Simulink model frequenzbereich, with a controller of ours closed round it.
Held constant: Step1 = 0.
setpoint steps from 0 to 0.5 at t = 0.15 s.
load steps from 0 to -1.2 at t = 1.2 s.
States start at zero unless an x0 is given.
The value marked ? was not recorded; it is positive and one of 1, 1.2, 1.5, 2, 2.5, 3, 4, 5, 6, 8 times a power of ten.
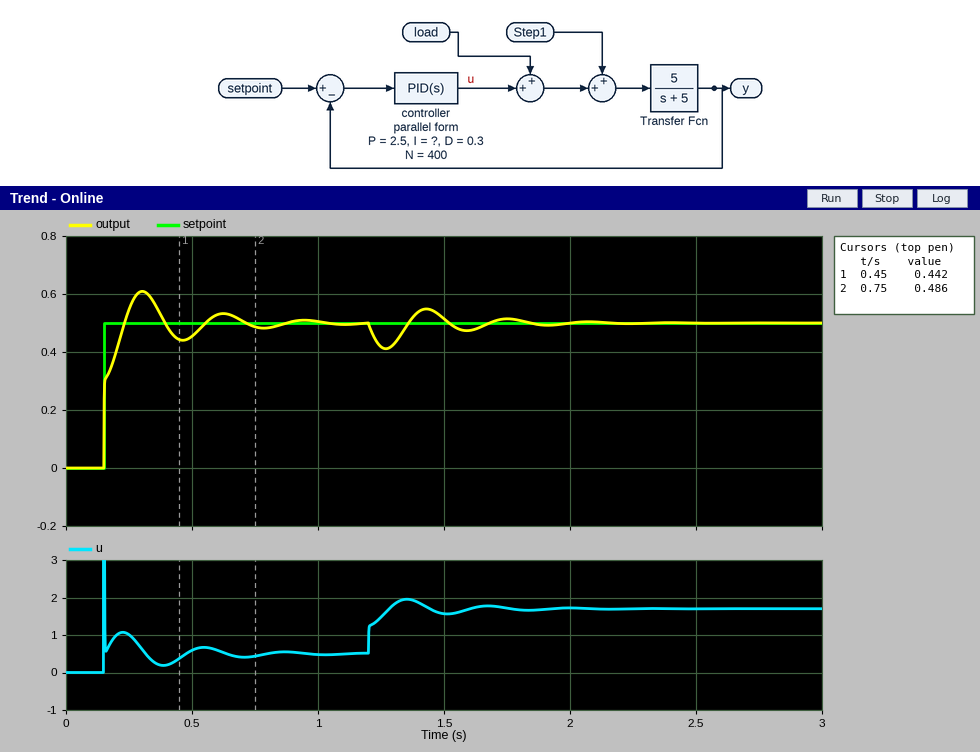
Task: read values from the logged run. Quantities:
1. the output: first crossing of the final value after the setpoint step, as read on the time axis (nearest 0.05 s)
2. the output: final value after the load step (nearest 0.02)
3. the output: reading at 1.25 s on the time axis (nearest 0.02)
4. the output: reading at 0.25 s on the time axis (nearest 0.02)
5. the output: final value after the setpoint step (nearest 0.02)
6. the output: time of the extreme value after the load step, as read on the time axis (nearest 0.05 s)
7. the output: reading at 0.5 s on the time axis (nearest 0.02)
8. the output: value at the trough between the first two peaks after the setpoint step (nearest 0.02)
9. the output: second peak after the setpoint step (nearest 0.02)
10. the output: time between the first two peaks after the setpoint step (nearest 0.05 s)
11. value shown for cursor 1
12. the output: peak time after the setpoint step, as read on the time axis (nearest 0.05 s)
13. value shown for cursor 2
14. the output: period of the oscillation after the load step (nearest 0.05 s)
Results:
0.25 s
0.50
0.42
0.54
0.50
1.25 s
0.46
0.44
0.54
0.30 s
0.442
0.30 s
0.486
0.30 s
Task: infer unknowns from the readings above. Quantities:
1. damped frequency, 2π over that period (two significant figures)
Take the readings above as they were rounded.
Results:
21 rad/s
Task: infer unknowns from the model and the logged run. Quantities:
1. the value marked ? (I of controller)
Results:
200
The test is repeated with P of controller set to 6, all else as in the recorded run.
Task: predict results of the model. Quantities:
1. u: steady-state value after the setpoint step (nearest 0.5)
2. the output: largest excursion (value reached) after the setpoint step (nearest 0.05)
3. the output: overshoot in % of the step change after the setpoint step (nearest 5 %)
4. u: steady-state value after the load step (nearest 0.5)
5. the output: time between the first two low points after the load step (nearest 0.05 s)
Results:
0.5
0.55
15 %
1.5
0.35 s
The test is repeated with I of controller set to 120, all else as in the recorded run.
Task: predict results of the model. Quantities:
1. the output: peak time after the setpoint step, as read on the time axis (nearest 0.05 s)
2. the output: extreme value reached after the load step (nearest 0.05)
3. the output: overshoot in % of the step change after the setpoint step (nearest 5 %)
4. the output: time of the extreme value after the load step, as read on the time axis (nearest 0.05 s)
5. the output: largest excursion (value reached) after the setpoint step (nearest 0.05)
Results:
0.35 s
0.40
20 %
1.30 s
0.60
